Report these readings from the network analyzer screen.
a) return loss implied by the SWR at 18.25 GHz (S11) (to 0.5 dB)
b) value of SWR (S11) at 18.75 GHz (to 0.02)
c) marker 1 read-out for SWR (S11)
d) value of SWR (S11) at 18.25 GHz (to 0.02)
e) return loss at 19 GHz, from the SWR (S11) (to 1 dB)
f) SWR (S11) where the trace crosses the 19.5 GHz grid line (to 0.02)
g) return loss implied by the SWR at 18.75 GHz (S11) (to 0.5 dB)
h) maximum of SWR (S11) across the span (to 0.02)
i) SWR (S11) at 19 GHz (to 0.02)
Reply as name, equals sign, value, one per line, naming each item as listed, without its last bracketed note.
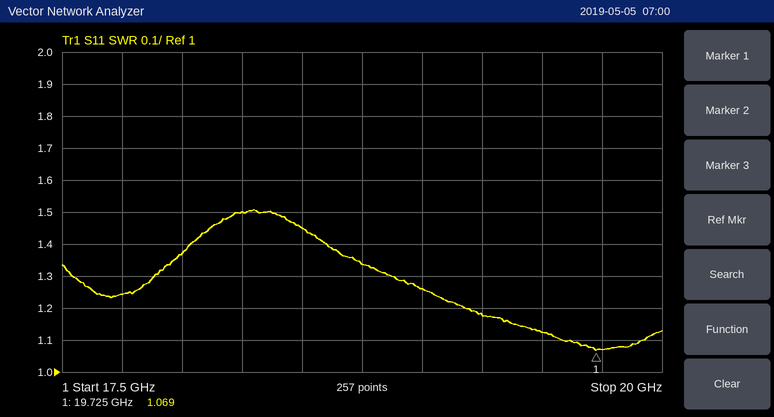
return loss implied by the SWR at 18.25 GHz (S11) = 14.0 dB
value of SWR (S11) at 18.75 GHz = 1.34
marker 1 read-out for SWR = 1.069
value of SWR (S11) at 18.25 GHz = 1.50
return loss at 19 GHz, from the SWR (S11) = 19 dB
SWR (S11) where the trace crosses the 19.5 GHz grid line = 1.12
return loss implied by the SWR at 18.75 GHz (S11) = 17.0 dB
maximum of SWR (S11) across the span = 1.50
SWR (S11) at 19 GHz = 1.26
